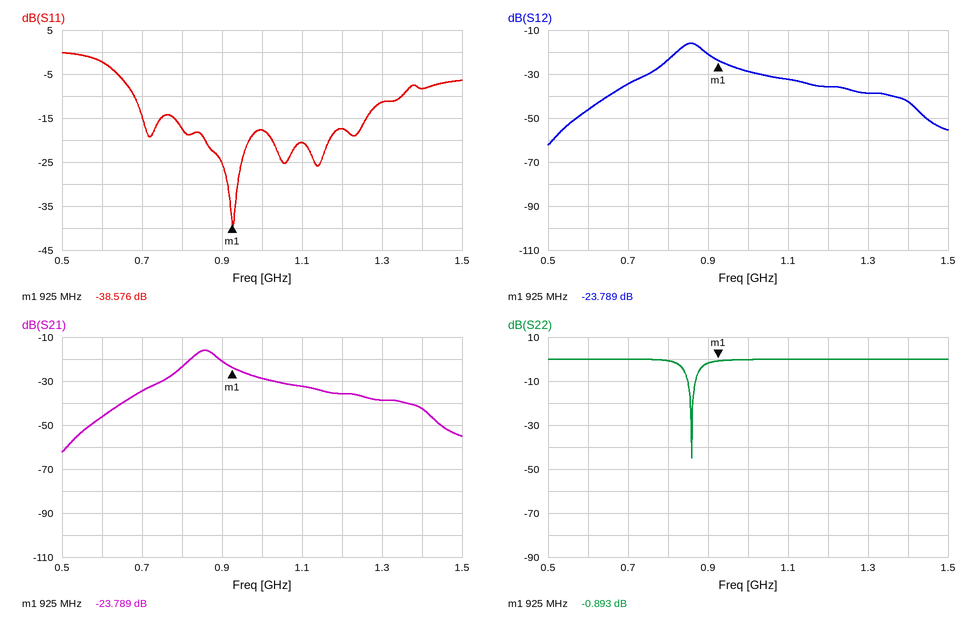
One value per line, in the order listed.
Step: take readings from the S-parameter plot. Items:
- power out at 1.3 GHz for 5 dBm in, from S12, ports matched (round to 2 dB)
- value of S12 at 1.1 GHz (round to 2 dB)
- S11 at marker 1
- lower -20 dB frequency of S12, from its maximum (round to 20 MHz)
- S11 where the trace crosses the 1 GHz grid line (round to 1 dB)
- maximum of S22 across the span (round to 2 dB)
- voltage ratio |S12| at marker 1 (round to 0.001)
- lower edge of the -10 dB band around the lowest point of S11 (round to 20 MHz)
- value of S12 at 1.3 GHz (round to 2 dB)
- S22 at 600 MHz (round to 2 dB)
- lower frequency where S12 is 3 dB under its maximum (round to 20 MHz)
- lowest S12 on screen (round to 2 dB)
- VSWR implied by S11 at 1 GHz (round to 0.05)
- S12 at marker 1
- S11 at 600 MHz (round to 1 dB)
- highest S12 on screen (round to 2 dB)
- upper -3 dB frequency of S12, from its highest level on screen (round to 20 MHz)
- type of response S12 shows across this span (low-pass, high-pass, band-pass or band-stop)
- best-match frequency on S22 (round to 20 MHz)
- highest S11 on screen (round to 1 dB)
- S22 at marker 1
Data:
-34 dBm
-32 dB
-38.576 dB
680 MHz
-18 dB
0 dB
0.065
680 MHz
-38 dB
0 dB
820 MHz
-62 dB
1.30
-23.789 dB
-2 dB
-16 dB
880 MHz
band-pass
860 MHz
0 dB
-0.893 dB
